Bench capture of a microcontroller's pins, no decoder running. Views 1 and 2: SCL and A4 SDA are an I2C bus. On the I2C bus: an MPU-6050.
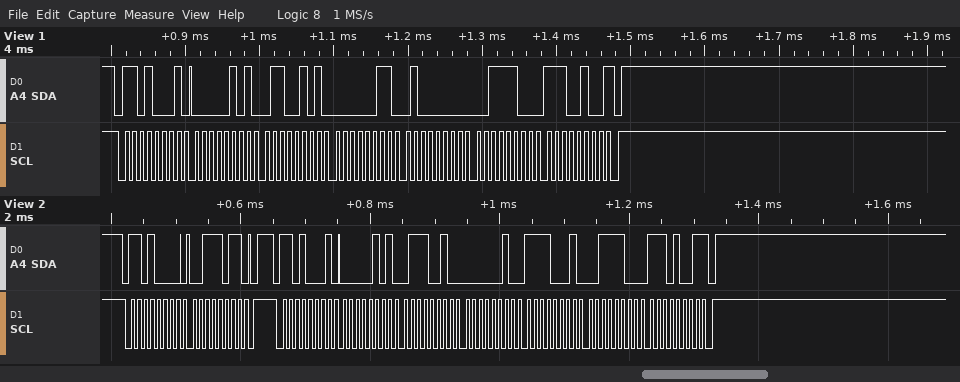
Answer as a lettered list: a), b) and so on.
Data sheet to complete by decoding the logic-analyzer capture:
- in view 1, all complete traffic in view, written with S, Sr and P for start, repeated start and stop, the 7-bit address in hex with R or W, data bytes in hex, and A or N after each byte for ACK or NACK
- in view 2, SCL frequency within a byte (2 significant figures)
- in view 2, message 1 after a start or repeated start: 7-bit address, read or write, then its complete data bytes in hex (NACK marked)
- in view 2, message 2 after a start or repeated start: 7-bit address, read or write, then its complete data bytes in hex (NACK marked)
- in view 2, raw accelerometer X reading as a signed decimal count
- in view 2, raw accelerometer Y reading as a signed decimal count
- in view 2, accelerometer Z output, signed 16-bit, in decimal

a) S 68R A 05 A 65 A 03 A 40 A 3C A E4 N P
b) 100 kHz
c) 0x68 write: 3B
d) 0x68 read: 05 72 02 F1 3C E9 NACK
e) 1394
f) 753
g) 15593
